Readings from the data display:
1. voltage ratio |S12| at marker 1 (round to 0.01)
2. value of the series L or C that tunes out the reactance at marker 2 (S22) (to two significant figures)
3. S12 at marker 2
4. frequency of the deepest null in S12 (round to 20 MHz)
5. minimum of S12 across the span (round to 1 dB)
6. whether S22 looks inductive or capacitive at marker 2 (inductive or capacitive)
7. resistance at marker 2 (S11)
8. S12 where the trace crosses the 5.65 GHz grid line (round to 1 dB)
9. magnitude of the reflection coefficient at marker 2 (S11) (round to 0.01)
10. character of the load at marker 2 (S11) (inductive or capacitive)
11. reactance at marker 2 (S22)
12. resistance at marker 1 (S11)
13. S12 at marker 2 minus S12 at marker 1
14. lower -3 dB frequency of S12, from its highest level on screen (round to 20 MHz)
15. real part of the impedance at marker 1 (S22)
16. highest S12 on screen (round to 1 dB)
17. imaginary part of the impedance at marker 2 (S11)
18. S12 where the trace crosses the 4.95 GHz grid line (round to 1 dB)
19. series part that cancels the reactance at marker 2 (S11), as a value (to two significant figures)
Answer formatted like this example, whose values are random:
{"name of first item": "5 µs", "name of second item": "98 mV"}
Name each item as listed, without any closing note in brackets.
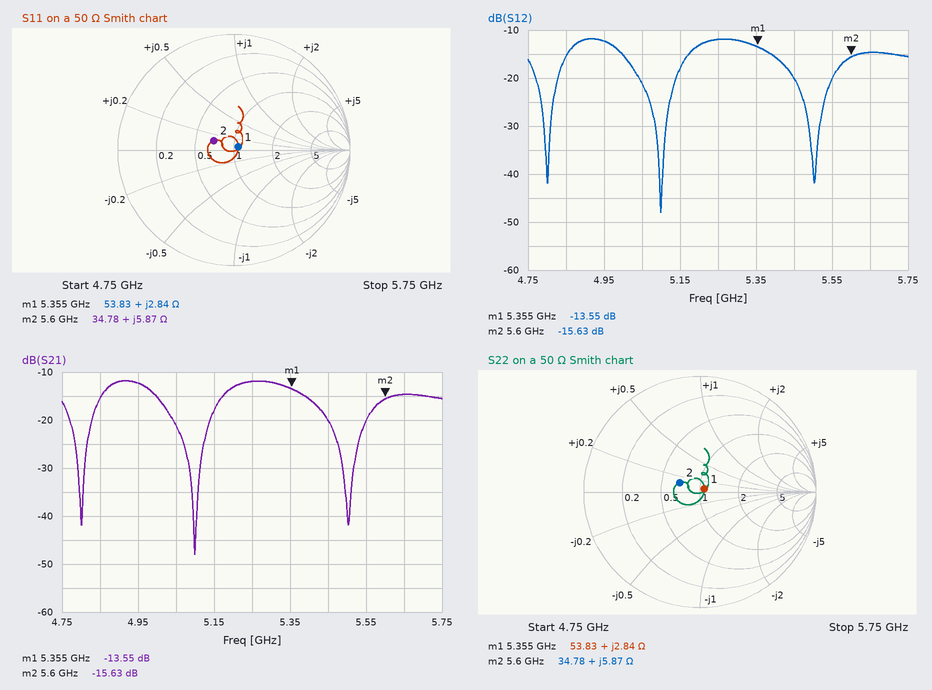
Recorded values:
{"voltage ratio |S12| at marker 1": "0.21", "value of the series L or C that tunes out the reactance at marker 2 (S22)": "4.8 pF", "S12 at marker 2": "-15.63 dB", "frequency of the deepest null in S12": "5.10 GHz", "minimum of S12 across the span": "-48 dB", "whether S22 looks inductive or capacitive at marker 2": "inductive", "resistance at marker 2": "34.78 Ω", "S12 where the trace crosses the 5.65 GHz grid line": "-15 dB", "magnitude of the reflection coefficient at marker 2 (S11)": "0.19", "character of the load at marker 2 (S11)": "inductive", "reactance at marker 2": "+5.87 Ω", "resistance at marker 1": "53.83 Ω", "S12 at marker 2 minus S12 at marker 1": "-2.08 dB", "lower -3 dB frequency of S12, from its highest level on screen": "4.86 GHz", "real part of the impedance at marker 1": "53.83 Ω", "highest S12 on screen": "-12 dB", "imaginary part of the impedance at marker 2": "+5.87 Ω", "S12 where the trace crosses the 4.95 GHz grid line": "-12 dB", "series part that cancels the reactance at marker 2 (S11), as a value": "4.8 pF"}
